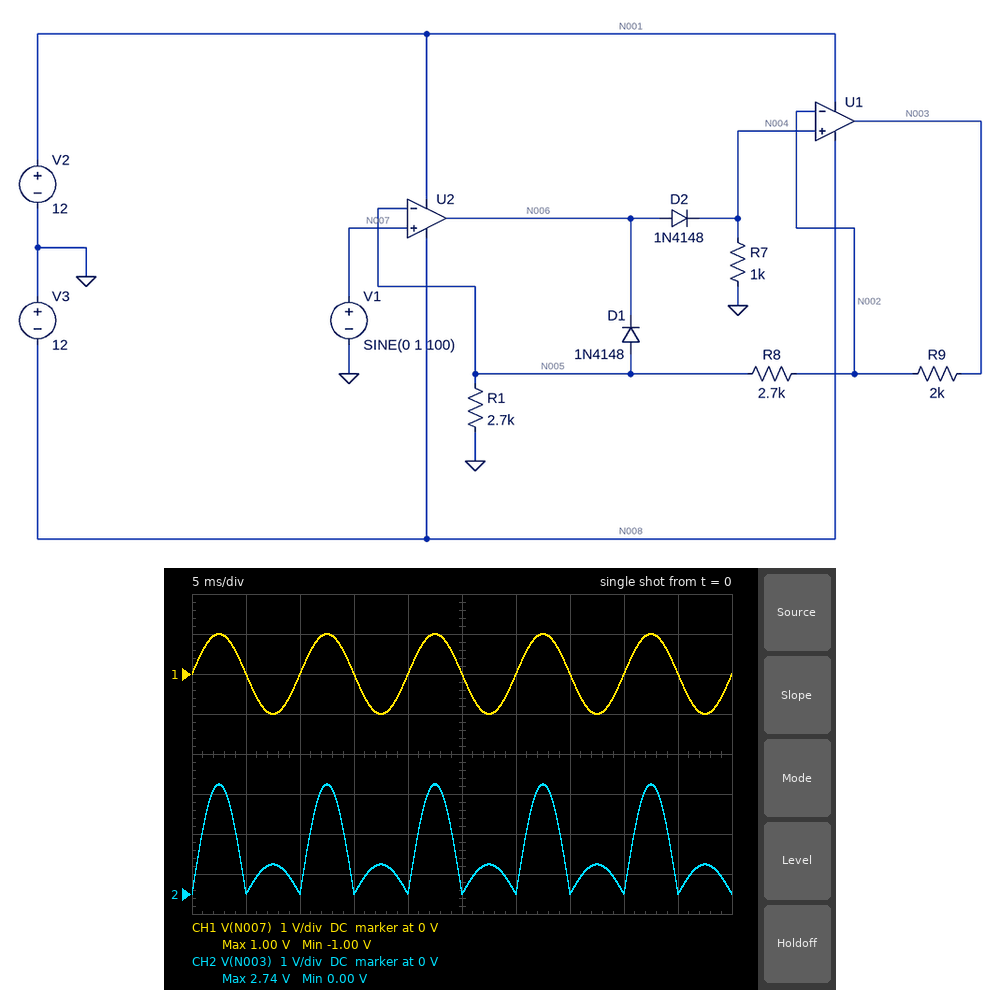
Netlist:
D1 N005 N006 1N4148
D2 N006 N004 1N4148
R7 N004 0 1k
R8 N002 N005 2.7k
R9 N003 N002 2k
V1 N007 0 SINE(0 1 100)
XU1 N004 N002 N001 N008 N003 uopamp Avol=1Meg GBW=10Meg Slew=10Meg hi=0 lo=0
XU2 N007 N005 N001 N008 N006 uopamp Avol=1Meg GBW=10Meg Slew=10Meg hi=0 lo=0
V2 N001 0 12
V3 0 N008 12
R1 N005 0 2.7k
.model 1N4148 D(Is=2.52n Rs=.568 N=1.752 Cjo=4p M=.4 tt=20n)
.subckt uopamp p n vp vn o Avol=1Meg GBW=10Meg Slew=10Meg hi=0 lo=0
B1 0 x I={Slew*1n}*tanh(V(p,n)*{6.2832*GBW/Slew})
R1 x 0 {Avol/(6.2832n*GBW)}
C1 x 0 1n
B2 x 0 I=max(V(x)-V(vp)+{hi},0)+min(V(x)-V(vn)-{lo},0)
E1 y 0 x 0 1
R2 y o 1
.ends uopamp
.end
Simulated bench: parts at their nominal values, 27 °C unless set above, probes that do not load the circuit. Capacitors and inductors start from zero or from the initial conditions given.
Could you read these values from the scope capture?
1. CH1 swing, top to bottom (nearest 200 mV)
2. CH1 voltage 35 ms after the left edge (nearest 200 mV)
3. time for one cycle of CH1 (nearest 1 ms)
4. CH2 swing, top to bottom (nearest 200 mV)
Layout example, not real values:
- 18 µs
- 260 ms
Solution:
- 2.0 V
- 0 V
- 10 ms
- 2.8 V
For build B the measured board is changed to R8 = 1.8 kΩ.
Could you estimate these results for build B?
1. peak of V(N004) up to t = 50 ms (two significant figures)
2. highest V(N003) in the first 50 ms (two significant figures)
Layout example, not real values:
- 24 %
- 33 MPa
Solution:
- 1.7 V
- 2.4 V
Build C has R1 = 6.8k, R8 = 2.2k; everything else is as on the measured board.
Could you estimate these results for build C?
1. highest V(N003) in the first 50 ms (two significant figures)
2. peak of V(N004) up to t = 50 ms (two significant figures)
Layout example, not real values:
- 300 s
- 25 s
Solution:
- 1.6 V
- 1.3 V
